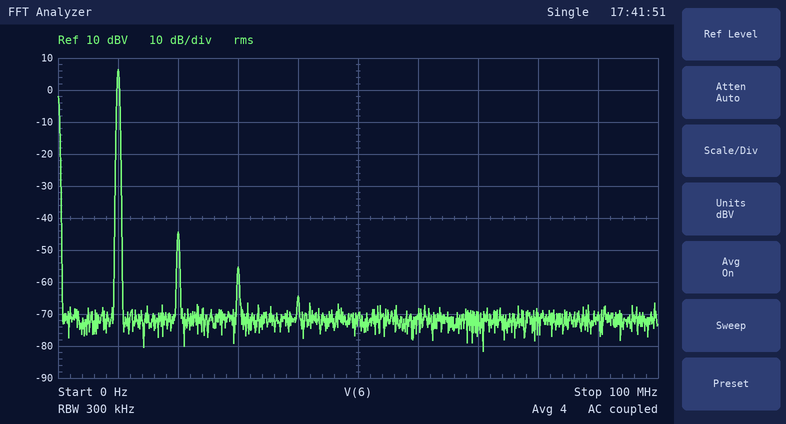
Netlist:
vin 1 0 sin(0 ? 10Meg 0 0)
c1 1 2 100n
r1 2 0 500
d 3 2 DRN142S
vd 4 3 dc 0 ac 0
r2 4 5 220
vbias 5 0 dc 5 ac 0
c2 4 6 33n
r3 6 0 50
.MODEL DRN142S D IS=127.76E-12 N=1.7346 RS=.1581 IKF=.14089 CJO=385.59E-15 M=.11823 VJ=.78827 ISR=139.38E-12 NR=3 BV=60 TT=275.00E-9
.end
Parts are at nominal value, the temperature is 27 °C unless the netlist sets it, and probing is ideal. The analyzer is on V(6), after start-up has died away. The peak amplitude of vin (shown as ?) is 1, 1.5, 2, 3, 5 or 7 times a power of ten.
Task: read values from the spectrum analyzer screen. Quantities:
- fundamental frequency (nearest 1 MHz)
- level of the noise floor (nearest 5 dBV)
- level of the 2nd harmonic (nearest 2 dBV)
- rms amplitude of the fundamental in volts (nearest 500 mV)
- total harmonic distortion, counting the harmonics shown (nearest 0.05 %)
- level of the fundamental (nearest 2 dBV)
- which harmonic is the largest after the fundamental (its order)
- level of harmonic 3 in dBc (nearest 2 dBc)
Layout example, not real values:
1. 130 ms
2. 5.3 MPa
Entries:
1. 10 MHz
2. -70 dBV
3. -44 dBV
4. 2.0 V
5. 0.30 %
6. 6 dBV
7. 2
8. -62 dBc
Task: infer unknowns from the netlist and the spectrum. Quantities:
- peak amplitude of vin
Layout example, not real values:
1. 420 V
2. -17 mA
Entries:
1. 3 V
